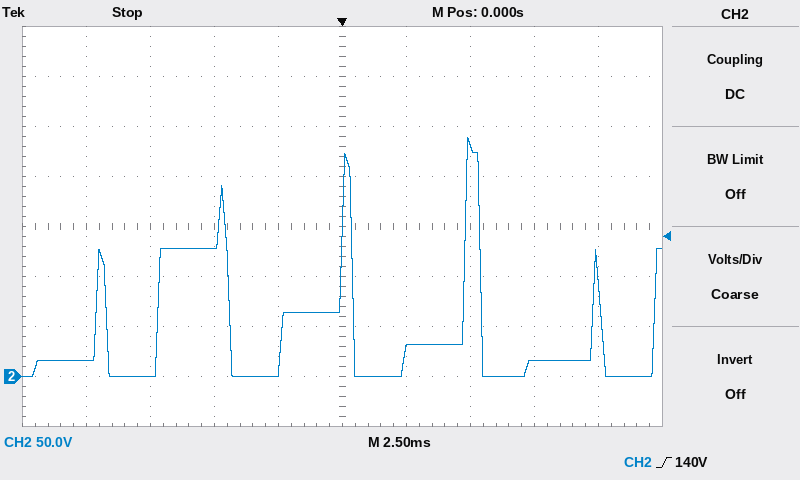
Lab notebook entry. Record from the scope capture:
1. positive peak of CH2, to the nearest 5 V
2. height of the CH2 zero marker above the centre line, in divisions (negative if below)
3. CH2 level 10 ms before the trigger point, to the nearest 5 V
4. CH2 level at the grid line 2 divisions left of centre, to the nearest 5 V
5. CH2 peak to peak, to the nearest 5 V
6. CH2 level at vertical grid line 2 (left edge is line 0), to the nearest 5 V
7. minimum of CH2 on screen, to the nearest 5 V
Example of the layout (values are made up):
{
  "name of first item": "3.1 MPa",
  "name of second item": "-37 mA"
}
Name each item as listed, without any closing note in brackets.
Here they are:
{
  "positive peak of CH2, to the nearest 5 V": "240 V",
  "height of the CH2 zero marker above the centre line, in divisions": "-3.0 div",
  "CH2 level 10 ms before the trigger point, to the nearest 5 V": "15 V",
  "CH2 level at the grid line 2 divisions left of centre, to the nearest 5 V": "130 V",
  "CH2 peak to peak, to the nearest 5 V": "240 V",
  "CH2 level at vertical grid line 2 (left edge is line 0), to the nearest 5 V": "0 V",
  "minimum of CH2 on screen, to the nearest 5 V": "0 V"
}
